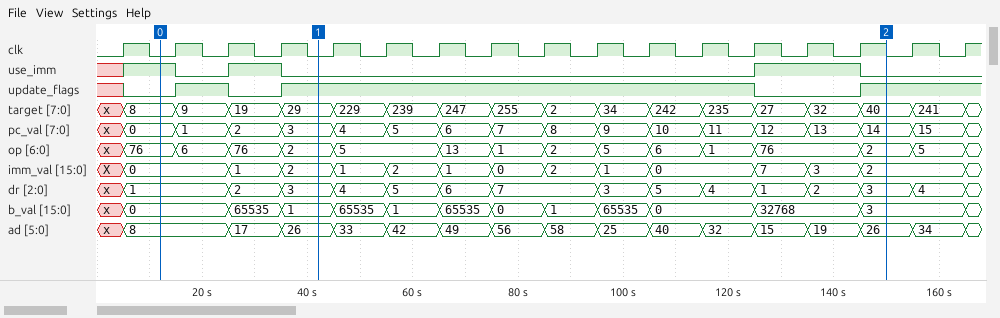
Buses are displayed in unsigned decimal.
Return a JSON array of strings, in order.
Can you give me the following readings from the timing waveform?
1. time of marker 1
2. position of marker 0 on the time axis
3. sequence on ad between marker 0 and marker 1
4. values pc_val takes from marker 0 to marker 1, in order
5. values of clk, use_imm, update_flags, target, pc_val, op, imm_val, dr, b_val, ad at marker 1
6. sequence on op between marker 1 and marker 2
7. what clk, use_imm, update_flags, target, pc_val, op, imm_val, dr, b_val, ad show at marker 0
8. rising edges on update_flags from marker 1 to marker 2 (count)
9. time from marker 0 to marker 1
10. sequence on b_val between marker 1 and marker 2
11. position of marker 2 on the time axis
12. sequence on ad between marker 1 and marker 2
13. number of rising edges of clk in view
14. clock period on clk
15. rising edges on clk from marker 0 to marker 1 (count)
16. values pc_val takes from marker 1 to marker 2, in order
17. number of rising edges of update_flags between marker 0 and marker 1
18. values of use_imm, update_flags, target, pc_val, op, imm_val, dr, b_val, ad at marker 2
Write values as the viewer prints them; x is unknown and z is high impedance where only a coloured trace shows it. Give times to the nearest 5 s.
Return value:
["40 s", "10 s", "8, 17, 26", "0, 1, 2, 3", "clk=0, use_imm=0, update_flags=1, target=29, pc_val=3, op=2, imm_val=2, dr=3, b_val=1, ad=26", "2, 5, 13, 1, 2, 5, 6, 1, 76, 2", "clk=0, use_imm=1, update_flags=0, target=8, pc_val=0, op=76, imm_val=0, dr=1, b_val=0, ad=8", "1", "30 s", "1, 65535, 1, 65535, 0, 1, 65535, 0, 32768, 3", "150 s", "26, 33, 42, 49, 56, 58, 25, 40, 32, 15, 19, 26", "17", "10 s", "3", "3, 4, 5, 6, 7, 8, 9, 10, 11, 12, 13, 14", "2", "use_imm=0, update_flags=1, target=40, pc_val=14, op=2, imm_val=2, dr=3, b_val=3, ad=26"]
